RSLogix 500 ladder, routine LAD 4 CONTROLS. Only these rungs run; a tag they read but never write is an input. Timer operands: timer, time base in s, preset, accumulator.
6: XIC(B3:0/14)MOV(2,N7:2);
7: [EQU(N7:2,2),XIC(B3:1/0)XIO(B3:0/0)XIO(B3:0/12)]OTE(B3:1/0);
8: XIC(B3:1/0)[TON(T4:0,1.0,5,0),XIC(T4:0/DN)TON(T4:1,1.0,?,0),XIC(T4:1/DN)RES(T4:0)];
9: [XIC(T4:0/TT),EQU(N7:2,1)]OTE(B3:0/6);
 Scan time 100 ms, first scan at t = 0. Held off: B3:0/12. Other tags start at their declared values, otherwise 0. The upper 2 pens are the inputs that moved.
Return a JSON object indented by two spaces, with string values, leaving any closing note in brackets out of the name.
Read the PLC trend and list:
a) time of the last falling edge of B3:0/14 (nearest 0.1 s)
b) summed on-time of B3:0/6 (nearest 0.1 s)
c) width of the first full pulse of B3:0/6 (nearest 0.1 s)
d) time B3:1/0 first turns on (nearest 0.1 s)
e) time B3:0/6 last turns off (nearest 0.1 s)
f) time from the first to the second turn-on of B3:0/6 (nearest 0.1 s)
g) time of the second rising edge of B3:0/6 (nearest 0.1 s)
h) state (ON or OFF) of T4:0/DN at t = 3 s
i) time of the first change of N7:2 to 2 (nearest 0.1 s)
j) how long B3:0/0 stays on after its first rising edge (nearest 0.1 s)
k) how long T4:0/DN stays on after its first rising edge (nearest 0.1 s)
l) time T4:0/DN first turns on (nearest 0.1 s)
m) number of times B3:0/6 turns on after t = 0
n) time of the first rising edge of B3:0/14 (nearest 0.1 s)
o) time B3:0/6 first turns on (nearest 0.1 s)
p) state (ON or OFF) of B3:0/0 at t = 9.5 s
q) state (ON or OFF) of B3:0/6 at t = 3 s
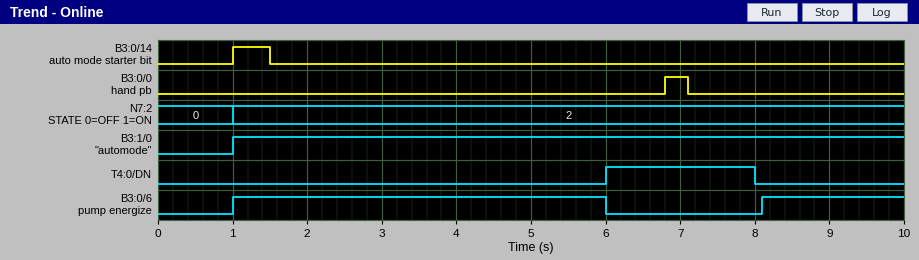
{
  "time of the last falling edge of B3:0/14": "1.5 s",
  "summed on-time of B3:0/6": "6.9 s",
  "width of the first full pulse of B3:0/6": "5.0 s",
  "time B3:1/0 first turns on": "1.0 s",
  "time B3:0/6 last turns off": "6.0 s",
  "time from the first to the second turn-on of B3:0/6": "7.1 s",
  "time of the second rising edge of B3:0/6": "8.1 s",
  "state (ON or OFF) of T4:0/DN at t = 3 s": "OFF",
  "time of the first change of N7:2 to 2": "1.0 s",
  "how long B3:0/0 stays on after its first rising edge": "0.3 s",
  "how long T4:0/DN stays on after its first rising edge": "2.0 s",
  "time T4:0/DN first turns on": "6.0 s",
  "number of times B3:0/6 turns on after t = 0": "2",
  "time of the first rising edge of B3:0/14": "1.0 s",
  "time B3:0/6 first turns on": "1.0 s",
  "state (ON or OFF) of B3:0/0 at t = 9.5 s": "OFF",
  "state (ON or OFF) of B3:0/6 at t = 3 s": "ON"
}
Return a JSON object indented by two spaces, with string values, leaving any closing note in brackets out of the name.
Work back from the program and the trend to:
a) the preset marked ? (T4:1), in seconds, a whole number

{
  "the preset marked ? (T4:1), in seconds, a whole number": "2 s"
}
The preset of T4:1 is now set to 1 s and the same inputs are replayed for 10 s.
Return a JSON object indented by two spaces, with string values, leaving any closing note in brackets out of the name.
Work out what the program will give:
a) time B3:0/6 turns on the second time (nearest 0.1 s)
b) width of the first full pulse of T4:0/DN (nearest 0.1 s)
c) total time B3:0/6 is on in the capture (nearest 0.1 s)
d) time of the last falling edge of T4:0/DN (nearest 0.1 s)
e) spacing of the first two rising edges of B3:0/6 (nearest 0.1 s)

{
  "time B3:0/6 turns on the second time": "7.1 s",
  "width of the first full pulse of T4:0/DN": "1.0 s",
  "total time B3:0/6 is on in the capture": "7.9 s",
  "time of the last falling edge of T4:0/DN": "7.0 s",
  "spacing of the first two rising edges of B3:0/6": "6.1 s"
}
